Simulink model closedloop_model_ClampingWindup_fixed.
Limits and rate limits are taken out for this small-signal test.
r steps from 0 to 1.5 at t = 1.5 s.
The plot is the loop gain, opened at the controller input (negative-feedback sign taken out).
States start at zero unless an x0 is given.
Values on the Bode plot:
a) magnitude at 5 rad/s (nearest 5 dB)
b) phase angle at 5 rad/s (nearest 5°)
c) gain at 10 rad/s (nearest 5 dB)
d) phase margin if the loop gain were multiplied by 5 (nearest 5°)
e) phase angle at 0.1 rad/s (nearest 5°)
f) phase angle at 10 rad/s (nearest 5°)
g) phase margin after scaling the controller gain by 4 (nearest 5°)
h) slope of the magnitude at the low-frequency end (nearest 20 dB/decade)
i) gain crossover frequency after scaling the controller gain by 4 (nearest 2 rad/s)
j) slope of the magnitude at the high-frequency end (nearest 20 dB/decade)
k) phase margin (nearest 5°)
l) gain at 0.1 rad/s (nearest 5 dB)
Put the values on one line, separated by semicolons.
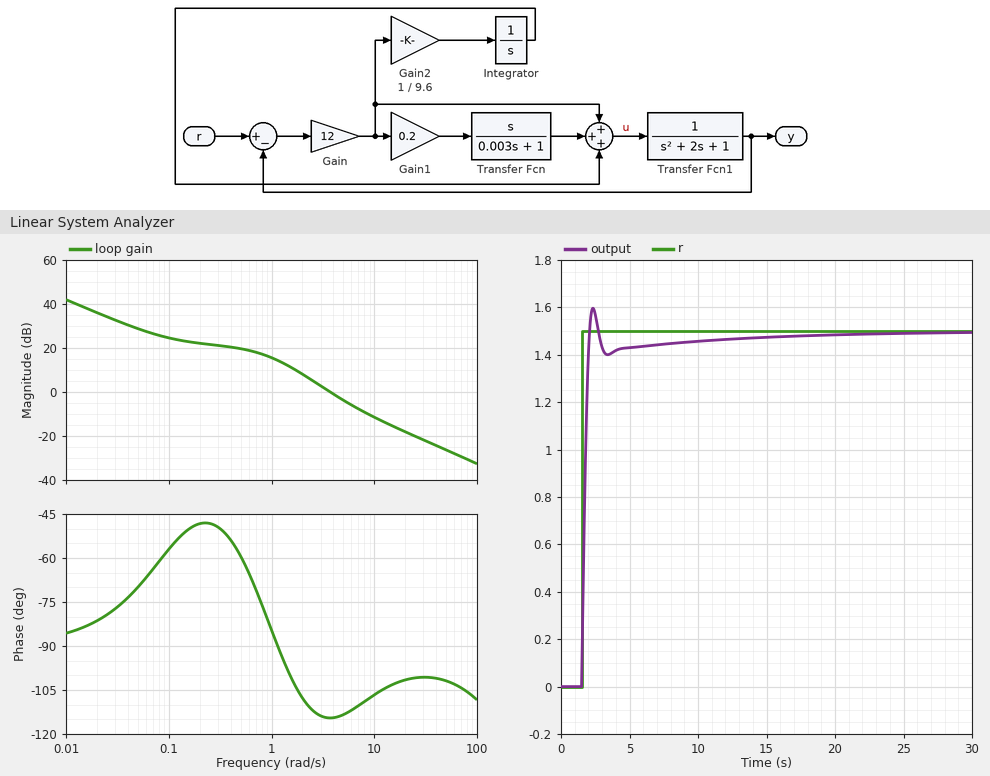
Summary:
-5 dB; -115°; -10 dB; 75°; -55°; -105°; 75°; -20 dB/decade; 10 rad/s; -20 dB/decade; 65°; 25 dB
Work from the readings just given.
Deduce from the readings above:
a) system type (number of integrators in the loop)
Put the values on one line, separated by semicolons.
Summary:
1
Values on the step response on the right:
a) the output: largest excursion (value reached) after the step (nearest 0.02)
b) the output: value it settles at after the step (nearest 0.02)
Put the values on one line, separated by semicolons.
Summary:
1.60; 1.50
